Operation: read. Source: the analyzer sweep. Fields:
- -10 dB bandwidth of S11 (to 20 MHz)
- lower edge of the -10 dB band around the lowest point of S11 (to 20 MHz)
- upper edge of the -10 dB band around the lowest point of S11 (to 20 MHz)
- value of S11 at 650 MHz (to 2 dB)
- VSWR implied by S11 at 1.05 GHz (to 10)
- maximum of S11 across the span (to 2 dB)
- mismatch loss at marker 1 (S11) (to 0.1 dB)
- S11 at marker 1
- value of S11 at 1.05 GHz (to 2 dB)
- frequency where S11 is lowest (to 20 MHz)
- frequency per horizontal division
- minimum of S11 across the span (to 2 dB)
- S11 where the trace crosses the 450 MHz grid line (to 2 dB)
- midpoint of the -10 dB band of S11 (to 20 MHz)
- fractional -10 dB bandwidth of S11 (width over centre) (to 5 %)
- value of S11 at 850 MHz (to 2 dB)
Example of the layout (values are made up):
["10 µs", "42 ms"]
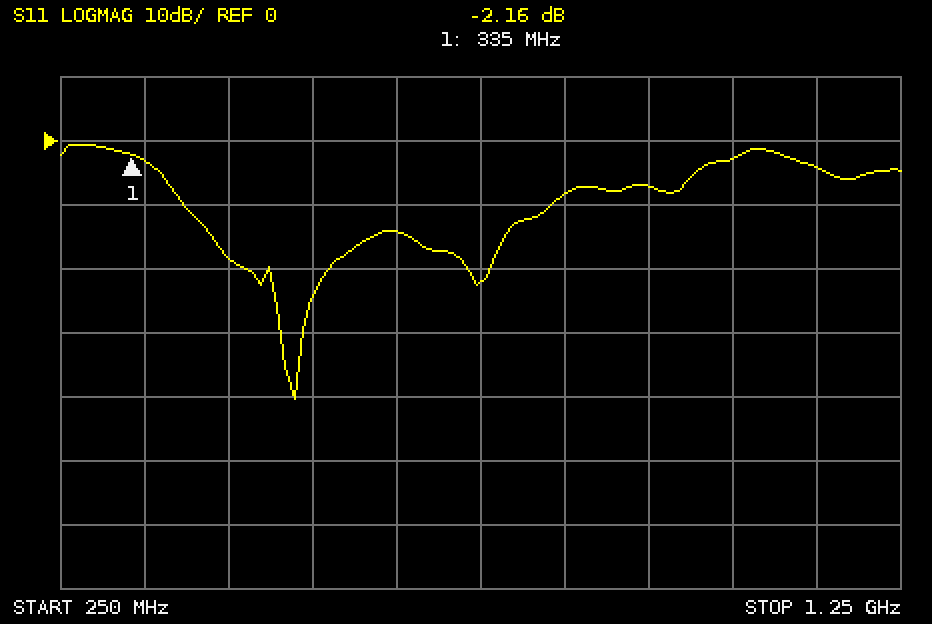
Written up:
["440 MHz", "400 MHz", "840 MHz", "-14 dB", "10", "0 dB", "4.1 dB", "-2.16 dB", "-2 dB", "520 MHz", "100 MHz", "-40 dB", "-18 dB", "620 MHz", "70 %", "-8 dB"]
